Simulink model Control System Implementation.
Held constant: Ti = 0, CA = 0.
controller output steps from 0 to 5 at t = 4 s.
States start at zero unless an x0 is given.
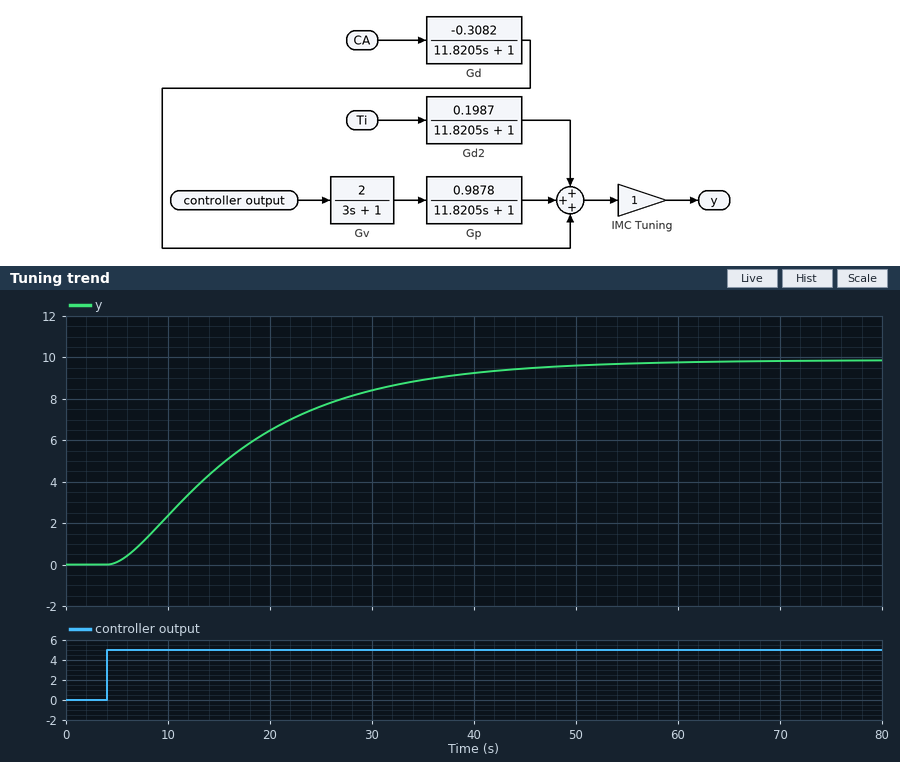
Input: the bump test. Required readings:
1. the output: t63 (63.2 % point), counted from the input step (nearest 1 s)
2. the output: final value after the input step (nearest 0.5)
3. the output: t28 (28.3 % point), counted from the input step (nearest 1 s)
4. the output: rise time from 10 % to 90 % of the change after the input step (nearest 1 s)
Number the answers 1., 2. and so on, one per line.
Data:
1. 15 s
2. 10.0
3. 7 s
4. 27 s
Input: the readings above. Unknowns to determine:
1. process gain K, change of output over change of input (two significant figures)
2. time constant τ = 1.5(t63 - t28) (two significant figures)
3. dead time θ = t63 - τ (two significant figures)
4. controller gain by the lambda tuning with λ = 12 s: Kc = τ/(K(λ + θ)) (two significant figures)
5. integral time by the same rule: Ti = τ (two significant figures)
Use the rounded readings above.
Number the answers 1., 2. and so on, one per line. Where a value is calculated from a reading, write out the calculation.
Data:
1. (10 - 0) / 5 = 2.0
2. 1.5 × (15 - 7) = 12 s
3. 15 - 12 = 3.0 s
4. 12 / (2 × (12 + 3)) = 0.40
5. 12 s
